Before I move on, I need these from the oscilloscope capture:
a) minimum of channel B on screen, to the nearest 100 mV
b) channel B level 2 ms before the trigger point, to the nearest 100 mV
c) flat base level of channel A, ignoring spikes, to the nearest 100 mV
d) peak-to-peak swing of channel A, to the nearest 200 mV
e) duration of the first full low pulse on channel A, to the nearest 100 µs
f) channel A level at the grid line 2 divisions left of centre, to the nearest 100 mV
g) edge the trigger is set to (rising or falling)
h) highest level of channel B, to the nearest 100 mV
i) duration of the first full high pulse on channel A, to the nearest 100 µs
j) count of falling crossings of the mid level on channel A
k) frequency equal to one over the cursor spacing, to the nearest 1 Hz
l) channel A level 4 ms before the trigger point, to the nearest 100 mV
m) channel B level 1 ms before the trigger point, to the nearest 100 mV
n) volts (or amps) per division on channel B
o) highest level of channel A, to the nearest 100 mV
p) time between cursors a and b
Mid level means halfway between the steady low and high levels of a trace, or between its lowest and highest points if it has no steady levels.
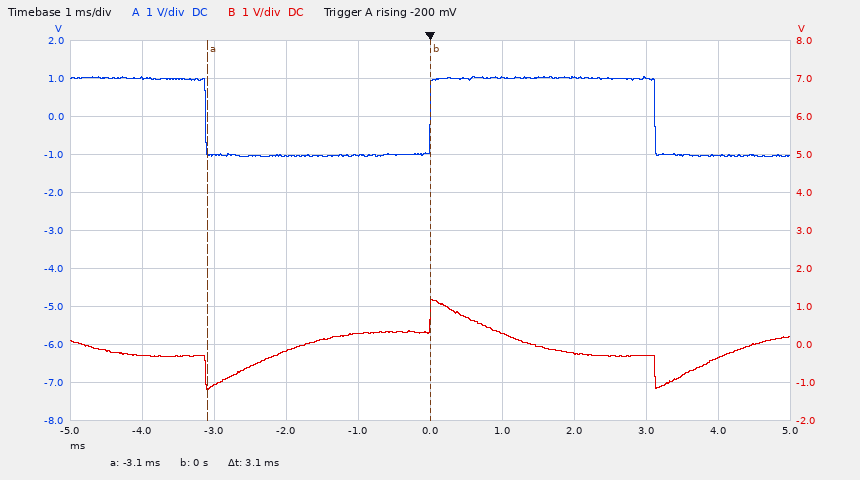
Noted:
-1.2 V
-200 mV
-1.0 V
2.2 V
3.1 ms
-1.0 V
rising
1.2 V
3.1 ms
2
323 Hz
1.0 V
300 mV
1 V
1.1 V
3.1 ms
